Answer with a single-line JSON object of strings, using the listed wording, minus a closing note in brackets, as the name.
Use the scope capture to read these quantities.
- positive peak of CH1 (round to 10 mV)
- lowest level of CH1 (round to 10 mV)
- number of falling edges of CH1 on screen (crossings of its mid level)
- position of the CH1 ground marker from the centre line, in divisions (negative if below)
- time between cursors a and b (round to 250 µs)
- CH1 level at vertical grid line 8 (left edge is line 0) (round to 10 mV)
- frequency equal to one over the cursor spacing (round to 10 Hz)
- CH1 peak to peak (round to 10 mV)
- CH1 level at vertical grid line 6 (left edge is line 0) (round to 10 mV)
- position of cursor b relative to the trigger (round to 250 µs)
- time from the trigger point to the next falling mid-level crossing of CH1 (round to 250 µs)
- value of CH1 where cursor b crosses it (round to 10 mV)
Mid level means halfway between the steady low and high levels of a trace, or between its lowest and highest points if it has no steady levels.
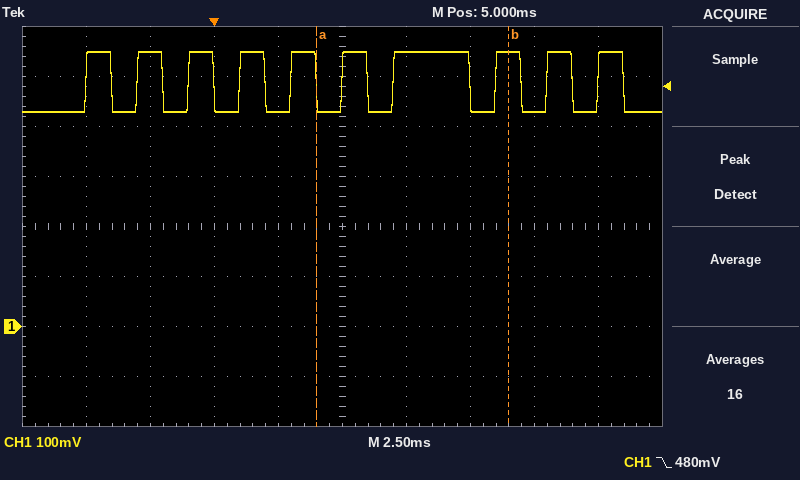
{"positive peak of CH1": "550 mV", "lowest level of CH1": "430 mV", "number of falling edges of CH1 on screen": "10", "position of the CH1 ground marker from the centre line, in divisions": "-2.0 div", "time between cursors a and b": "7.50 ms", "CH1 level at vertical grid line 8 (left edge is line 0)": "430 mV", "frequency equal to one over the cursor spacing": "130 Hz", "CH1 peak to peak": "120 mV", "CH1 level at vertical grid line 6 (left edge is line 0)": "550 mV", "position of cursor b relative to the trigger": "+11.50 ms", "time from the trigger point to the next falling mid-level crossing of CH1": "2.00 ms", "value of CH1 where cursor b crosses it": "550 mV"}
